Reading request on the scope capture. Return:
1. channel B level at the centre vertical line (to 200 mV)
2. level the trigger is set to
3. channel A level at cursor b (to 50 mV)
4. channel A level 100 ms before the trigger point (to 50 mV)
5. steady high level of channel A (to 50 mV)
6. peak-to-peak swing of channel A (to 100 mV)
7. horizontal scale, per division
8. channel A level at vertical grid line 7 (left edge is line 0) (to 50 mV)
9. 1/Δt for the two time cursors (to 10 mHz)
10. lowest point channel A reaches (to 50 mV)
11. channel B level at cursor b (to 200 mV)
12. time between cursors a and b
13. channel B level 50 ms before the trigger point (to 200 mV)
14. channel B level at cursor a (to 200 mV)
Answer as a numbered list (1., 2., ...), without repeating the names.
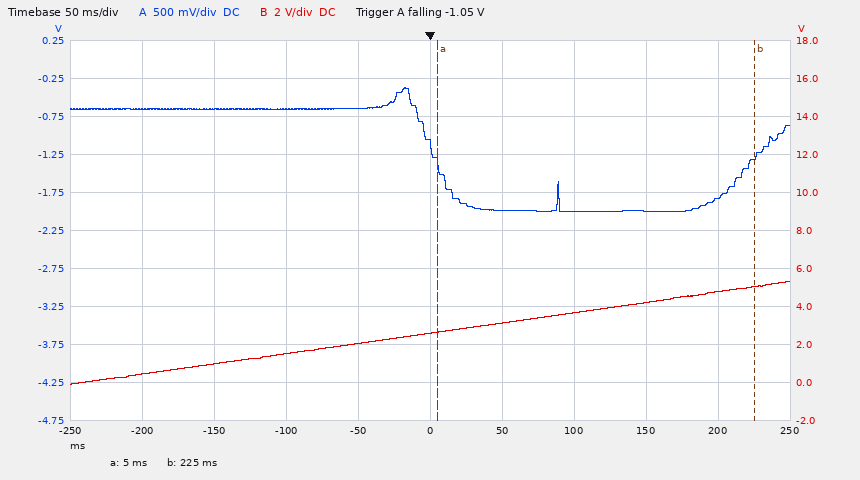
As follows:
1. 2.6 V
2. -1.05 V
3. -1.25 V
4. -650 mV
5. -650 mV
6. 1.60 V
7. 50 ms
8. -2.00 V
9. 4.55 Hz
10. -2.00 V
11. 5.0 V
12. 220 ms
13. 2.0 V
14. 2.6 V
